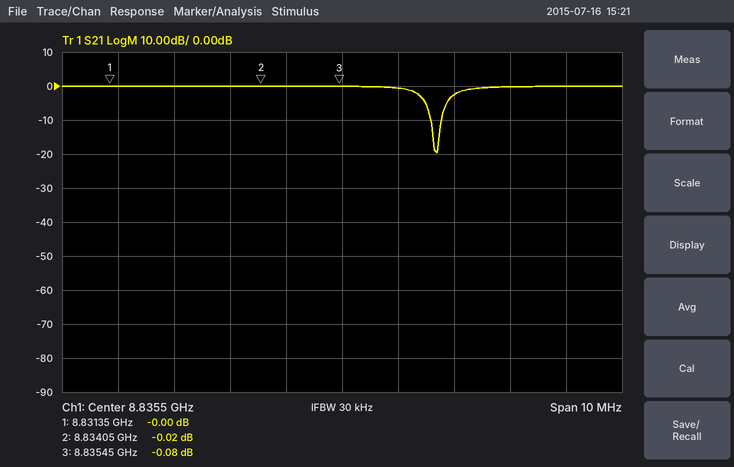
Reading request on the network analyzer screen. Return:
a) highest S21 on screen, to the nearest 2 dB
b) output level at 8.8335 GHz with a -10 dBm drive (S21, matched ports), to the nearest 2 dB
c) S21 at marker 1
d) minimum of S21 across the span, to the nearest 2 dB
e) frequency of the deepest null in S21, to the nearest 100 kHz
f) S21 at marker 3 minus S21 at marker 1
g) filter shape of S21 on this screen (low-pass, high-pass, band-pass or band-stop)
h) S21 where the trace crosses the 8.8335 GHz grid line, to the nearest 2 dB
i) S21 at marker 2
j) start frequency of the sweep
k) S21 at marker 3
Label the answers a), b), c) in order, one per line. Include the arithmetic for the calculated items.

a) 0 dB
b) -10 dBm + (0 dB) = -10 dBm
c) -0.00 dB
d) -20 dB
e) 8.8372 GHz
f) -0.08 − (-0) = -0.08 dB
g) band-stop
h) 0 dB
i) -0.02 dB
j) 8.8305 GHz
k) -0.08 dB
